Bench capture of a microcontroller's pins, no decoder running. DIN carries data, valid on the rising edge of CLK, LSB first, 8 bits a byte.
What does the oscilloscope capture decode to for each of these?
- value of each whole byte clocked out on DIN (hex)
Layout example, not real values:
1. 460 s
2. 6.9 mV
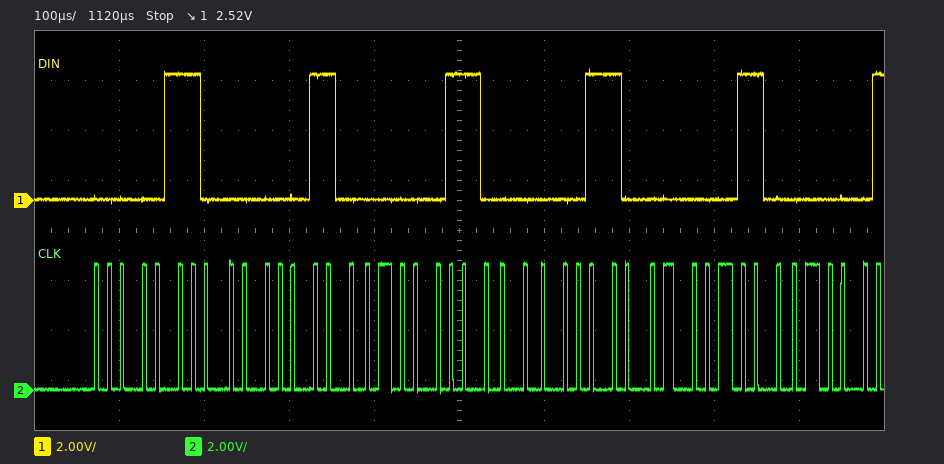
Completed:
1. 60 60 60 60 60
